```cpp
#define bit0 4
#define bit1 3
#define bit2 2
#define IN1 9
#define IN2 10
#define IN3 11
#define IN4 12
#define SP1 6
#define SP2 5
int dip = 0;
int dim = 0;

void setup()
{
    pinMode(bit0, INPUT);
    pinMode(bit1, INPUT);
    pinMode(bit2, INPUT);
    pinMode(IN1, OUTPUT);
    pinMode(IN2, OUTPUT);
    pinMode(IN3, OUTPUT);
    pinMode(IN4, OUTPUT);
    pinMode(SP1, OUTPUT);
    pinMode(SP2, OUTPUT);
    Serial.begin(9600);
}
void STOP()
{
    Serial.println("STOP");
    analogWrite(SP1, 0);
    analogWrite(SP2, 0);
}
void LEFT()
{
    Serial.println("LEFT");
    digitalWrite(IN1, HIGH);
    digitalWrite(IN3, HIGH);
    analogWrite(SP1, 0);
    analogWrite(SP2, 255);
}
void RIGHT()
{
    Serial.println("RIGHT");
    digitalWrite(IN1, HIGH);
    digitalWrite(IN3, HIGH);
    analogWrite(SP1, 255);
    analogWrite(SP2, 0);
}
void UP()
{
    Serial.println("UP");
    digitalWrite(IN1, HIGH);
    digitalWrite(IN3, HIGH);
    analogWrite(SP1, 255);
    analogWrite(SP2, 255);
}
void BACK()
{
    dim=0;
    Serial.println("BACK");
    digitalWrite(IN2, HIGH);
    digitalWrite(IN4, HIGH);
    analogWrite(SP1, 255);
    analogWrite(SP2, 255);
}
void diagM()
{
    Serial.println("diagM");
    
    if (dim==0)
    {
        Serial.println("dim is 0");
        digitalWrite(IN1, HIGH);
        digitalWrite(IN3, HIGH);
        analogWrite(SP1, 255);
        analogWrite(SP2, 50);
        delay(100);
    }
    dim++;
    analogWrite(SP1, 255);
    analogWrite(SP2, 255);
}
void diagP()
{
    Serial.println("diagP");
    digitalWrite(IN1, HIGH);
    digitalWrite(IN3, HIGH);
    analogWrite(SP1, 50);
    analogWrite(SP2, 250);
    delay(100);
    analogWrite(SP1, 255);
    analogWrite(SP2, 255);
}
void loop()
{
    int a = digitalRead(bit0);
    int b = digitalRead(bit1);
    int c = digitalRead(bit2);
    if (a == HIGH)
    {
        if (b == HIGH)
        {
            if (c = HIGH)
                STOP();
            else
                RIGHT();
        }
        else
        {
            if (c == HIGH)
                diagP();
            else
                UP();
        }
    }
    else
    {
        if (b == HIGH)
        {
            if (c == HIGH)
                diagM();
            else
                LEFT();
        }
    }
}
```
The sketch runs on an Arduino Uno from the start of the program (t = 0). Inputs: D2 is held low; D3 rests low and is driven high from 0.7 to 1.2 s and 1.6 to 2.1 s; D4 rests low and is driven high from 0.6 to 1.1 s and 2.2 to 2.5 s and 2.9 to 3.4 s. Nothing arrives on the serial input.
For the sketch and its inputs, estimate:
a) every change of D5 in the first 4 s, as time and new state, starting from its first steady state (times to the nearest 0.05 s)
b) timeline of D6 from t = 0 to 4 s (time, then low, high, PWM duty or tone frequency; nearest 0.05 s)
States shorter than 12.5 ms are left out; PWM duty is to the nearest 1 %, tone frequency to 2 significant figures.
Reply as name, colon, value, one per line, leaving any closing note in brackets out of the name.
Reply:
every change of D5 in the first 4 s, as time and new state, starting from its first steady state: 0 s low; 0.6 s high; 0.7 s low; 1.1 s high
timeline of D6 from t = 0 to 4 s: 0 s low; 0.6 s high; 0.7 s low; 2.2 s high
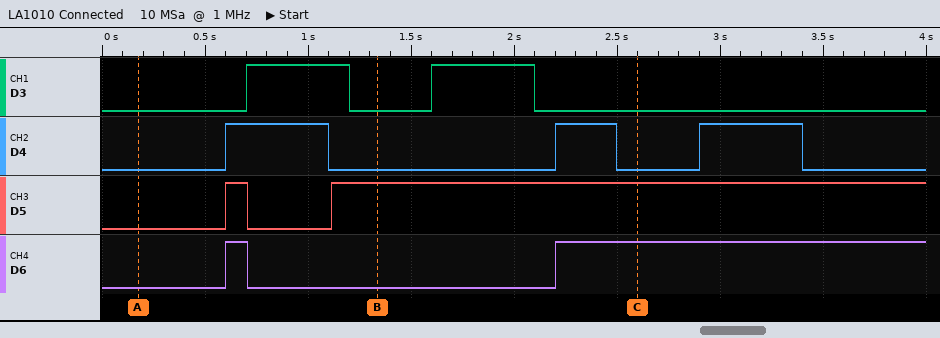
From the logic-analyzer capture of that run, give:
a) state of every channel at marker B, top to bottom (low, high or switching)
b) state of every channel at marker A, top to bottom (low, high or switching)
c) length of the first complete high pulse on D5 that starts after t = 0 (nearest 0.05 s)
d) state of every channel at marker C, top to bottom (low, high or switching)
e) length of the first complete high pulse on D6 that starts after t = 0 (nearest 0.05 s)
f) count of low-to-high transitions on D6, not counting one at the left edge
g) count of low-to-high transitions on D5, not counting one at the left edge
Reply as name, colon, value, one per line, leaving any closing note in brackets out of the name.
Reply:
state of every channel at marker B, top to bottom: D3 low, D4 low, D5 high, D6 low
state of every channel at marker A, top to bottom: D3 low, D4 low, D5 low, D6 low
length of the first complete high pulse on D5 that starts after t = 0: 0.10 s
state of every channel at marker C, top to bottom: D3 low, D4 low, D5 high, D6 high
length of the first complete high pulse on D6 that starts after t = 0: 0.10 s
count of low-to-high transitions on D6, not counting one at the left edge: 2
count of low-to-high transitions on D5, not counting one at the left edge: 2
